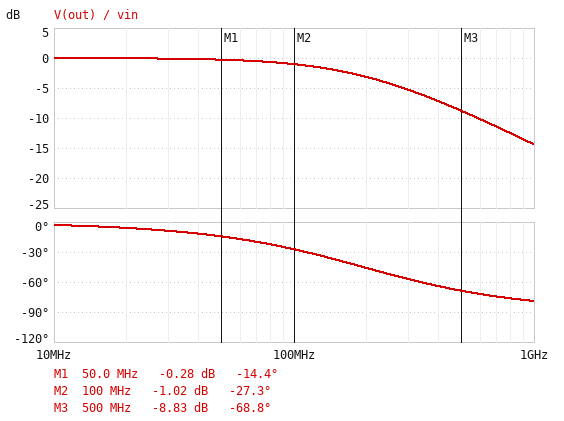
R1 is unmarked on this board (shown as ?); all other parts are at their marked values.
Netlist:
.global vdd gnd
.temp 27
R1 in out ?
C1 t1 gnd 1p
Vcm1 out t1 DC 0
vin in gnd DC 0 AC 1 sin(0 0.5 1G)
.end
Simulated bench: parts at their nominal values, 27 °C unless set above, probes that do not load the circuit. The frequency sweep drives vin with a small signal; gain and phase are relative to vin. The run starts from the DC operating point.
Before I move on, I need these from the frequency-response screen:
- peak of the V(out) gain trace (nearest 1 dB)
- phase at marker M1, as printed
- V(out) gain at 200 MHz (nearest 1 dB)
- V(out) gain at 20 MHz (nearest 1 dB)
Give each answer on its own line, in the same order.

0 dB
-14.4 deg
-3 dB
0 dB
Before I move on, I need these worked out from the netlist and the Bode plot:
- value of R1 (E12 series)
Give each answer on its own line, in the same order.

820 Ω
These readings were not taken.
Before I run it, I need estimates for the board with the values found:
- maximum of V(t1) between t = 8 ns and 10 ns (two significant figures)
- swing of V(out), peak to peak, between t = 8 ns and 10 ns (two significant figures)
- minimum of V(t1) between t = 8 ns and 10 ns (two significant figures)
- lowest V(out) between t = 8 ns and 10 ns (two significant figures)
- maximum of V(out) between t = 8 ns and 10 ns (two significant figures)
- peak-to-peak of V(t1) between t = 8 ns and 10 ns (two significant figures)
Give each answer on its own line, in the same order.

95 mV
190 mV
-95 mV
-95 mV
95 mV
190 mV
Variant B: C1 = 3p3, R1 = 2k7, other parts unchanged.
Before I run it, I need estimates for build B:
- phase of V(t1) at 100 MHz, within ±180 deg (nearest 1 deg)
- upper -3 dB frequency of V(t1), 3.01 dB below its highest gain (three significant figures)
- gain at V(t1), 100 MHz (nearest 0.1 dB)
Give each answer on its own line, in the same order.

-80 deg
17.9 MHz
-15.1 dB
